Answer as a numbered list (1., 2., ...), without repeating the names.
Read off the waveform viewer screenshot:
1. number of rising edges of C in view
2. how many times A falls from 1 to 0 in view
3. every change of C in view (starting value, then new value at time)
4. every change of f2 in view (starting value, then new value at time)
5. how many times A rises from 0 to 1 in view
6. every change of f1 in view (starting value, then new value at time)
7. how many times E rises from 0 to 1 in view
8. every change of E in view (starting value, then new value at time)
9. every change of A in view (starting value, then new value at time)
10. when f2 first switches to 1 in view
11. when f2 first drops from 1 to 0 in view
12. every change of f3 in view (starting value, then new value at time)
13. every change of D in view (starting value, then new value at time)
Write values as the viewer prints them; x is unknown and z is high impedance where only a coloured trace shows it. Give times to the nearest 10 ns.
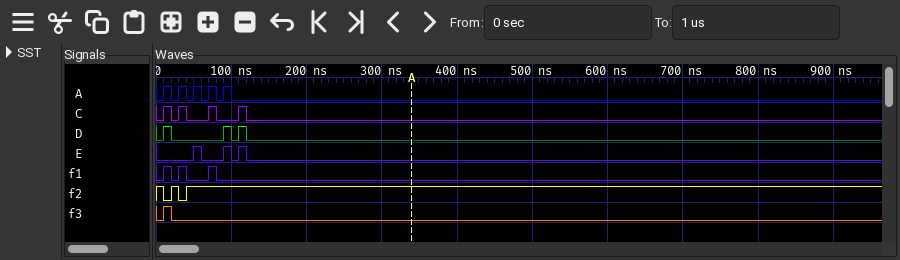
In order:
1. 4
2. 5
3. 0, 1 at 10 ns, 0 at 20 ns, 1 at 30 ns, 0 at 40 ns, 1 at 70 ns, 0 at 80 ns, 1 at 110 ns, 0 at 120 ns
4. 1, 0 at 10 ns, 1 at 20 ns, 0 at 30 ns, 1 at 40 ns
5. 5
6. 0, 1 at 10 ns, 0 at 20 ns, 1 at 30 ns, 0 at 40 ns, 1 at 70 ns, 0 at 80 ns
7. 3
8. 0, 1 at 50 ns, 0 at 60 ns, 1 at 90 ns, 0 at 100 ns, 1 at 110 ns, 0 at 120 ns
9. 0, 1 at 10 ns, 0 at 20 ns, 1 at 30 ns, 0 at 40 ns, 1 at 50 ns, 0 at 60 ns, 1 at 70 ns, 0 at 80 ns, 1 at 90 ns, 0 at 100 ns
10. 20 ns
11. 10 ns
12. 0, 1 at 10 ns, 0 at 20 ns
13. 0, 1 at 10 ns, 0 at 20 ns, 1 at 90 ns, 0 at 100 ns, 1 at 110 ns, 0 at 120 ns
